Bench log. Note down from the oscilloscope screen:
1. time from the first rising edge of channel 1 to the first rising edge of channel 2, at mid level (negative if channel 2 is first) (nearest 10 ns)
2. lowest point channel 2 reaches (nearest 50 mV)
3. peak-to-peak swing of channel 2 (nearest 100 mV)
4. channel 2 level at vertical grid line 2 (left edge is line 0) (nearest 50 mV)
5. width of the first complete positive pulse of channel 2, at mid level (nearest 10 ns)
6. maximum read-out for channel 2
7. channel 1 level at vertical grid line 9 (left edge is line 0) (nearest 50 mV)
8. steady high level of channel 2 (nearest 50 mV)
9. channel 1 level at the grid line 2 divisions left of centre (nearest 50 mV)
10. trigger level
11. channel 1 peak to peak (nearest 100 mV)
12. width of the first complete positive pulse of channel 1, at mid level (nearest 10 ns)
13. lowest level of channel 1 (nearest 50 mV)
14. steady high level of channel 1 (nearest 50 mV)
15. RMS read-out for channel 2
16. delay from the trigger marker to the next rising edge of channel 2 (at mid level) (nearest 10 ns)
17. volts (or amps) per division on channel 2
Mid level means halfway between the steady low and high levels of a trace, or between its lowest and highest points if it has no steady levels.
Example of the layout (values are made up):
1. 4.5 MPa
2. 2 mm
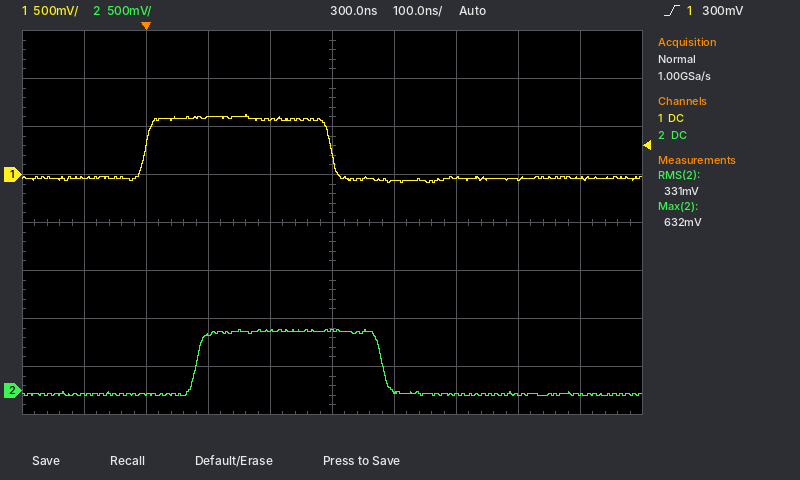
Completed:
1. +80 ns
2. -50 mV
3. 700 mV
4. -50 mV
5. 300 ns
6. 632 mV
7. -50 mV
8. 600 mV
9. 600 mV
10. 300 mV
11. 700 mV
12. 300 ns
13. -100 mV
14. 600 mV
15. 331 mV
16. 80 ns
17. 500 mV
